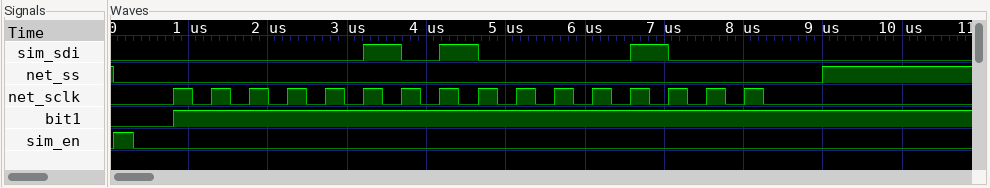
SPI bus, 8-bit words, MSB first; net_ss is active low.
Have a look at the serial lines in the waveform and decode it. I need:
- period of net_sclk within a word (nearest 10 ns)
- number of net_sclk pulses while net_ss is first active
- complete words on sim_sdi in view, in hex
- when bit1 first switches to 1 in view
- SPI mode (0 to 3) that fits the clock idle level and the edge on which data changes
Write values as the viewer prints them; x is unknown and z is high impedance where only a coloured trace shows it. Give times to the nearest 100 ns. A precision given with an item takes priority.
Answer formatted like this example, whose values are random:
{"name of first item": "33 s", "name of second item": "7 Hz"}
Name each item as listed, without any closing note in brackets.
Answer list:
{"period of net_sclk within a word": "480 ns", "number of net_sclk pulses while net_ss is first active": "16", "complete words on sim_sdi in view, in hex": "05, 08", "when bit1 first switches to 1 in view": "800 ns", "SPI mode (0 to 3) that fits the clock idle level and the edge on which data changes": "1"}
